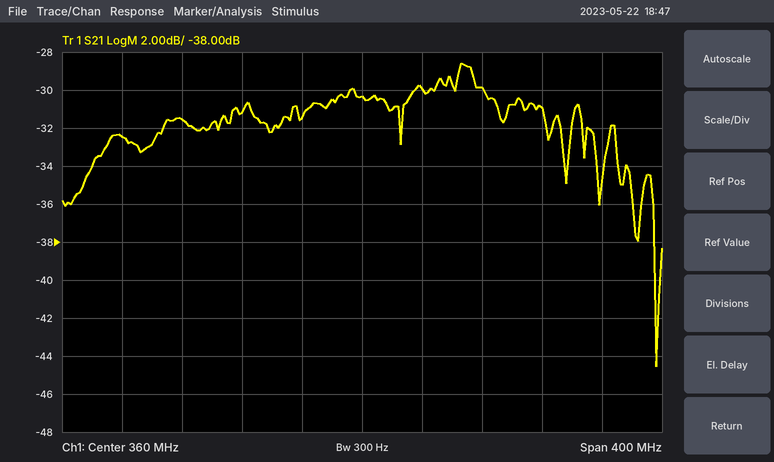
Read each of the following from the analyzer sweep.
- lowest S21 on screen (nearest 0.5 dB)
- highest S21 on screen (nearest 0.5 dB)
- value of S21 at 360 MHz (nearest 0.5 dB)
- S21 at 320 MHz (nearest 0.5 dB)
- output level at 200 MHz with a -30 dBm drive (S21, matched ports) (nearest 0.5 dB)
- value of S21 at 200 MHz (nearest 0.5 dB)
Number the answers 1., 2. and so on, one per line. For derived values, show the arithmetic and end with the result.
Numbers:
1. -44.5 dB
2. -28.5 dB
3. -30.5 dB
4. -31.5 dB
5. -30 dBm + (-32.5 dB) = -62.5 dBm
6. -32.5 dB
